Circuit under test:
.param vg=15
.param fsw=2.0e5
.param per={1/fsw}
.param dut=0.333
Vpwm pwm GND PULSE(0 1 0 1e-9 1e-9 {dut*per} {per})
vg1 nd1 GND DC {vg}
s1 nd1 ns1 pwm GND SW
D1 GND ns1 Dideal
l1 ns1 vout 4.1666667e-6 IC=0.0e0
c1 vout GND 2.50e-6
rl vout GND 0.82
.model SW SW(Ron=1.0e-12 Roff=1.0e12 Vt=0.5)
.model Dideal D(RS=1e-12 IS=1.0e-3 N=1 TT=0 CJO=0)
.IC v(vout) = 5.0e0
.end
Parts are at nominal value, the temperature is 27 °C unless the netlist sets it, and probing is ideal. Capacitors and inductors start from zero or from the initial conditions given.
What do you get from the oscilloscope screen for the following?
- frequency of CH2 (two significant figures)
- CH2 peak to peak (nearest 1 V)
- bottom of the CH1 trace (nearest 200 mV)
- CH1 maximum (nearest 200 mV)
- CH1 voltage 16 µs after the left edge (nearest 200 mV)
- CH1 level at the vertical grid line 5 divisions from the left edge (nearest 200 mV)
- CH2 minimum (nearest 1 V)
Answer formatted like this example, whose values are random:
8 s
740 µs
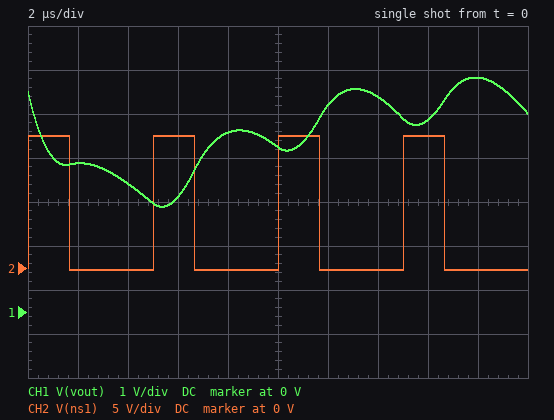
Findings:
200 kHz
15 V
2.4 V
5.4 V
4.4 V
3.8 V
0 V
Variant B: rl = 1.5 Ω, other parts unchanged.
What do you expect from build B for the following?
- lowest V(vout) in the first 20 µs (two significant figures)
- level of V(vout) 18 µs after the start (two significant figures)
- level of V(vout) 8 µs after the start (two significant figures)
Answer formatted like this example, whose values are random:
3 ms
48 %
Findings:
3.4 V
5.5 V
4.7 V
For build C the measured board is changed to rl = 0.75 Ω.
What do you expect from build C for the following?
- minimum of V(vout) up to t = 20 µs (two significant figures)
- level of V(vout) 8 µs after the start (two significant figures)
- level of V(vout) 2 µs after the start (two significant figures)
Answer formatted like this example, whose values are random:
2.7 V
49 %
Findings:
2.3 V
4.0 V
3.2 V
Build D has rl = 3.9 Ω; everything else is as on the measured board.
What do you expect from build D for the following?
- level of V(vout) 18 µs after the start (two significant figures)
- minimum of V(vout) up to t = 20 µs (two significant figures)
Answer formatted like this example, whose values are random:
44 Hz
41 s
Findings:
6.5 V
4.9 V
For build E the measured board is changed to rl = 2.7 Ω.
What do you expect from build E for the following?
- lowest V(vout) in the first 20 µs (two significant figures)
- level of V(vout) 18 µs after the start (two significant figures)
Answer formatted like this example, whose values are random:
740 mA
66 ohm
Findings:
4.6 V
5.7 V
